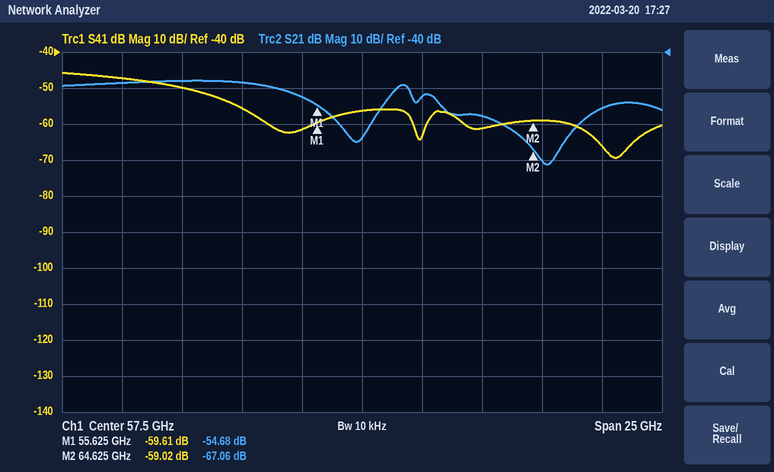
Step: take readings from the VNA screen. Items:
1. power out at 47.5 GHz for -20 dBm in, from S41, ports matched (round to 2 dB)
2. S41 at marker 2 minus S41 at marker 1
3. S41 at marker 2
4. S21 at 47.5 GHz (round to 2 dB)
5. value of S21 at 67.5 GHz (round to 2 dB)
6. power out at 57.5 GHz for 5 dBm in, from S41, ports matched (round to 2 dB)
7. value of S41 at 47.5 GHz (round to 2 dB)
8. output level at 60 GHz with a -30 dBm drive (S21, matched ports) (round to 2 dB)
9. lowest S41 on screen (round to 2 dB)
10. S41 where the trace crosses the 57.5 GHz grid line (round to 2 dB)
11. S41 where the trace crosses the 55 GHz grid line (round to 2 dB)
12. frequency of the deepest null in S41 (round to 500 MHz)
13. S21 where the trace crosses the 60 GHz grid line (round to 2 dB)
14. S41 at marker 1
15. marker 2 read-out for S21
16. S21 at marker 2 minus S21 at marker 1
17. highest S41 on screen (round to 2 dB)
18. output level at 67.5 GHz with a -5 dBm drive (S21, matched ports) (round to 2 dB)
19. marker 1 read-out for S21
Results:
-68 dBm
0.59 dB
-59.02 dB
-48 dB
-56 dB
-52 dBm
-48 dB
-82 dBm
-70 dB
-56 dB
-62 dB
68.0 GHz
-52 dB
-59.61 dB
-67.06 dB
-12.38 dB
-46 dB
-60 dBm
-54.68 dB
